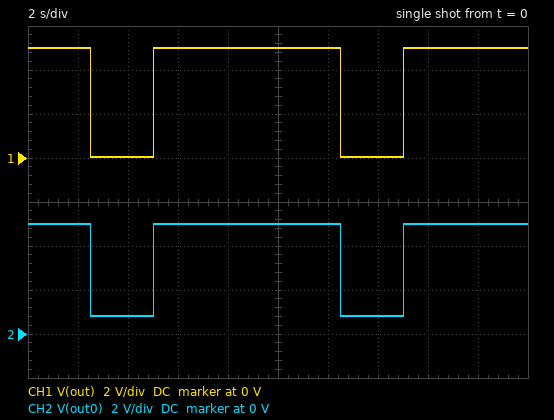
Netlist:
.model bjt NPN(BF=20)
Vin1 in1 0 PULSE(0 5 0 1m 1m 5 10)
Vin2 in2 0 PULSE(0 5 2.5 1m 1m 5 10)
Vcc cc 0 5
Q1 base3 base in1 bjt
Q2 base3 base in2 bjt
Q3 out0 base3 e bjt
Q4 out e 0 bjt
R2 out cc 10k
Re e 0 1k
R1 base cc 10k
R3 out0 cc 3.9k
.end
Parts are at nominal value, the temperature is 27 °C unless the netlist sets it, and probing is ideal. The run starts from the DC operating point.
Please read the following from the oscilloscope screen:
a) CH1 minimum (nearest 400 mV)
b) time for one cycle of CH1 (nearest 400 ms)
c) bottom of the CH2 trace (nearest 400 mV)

0 V
10.0 s
800 mV
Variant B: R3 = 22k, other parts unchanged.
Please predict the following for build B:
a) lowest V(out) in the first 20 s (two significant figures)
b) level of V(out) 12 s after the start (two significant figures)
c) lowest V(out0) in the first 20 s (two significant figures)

2.8 V
5.0 V
720 mV
